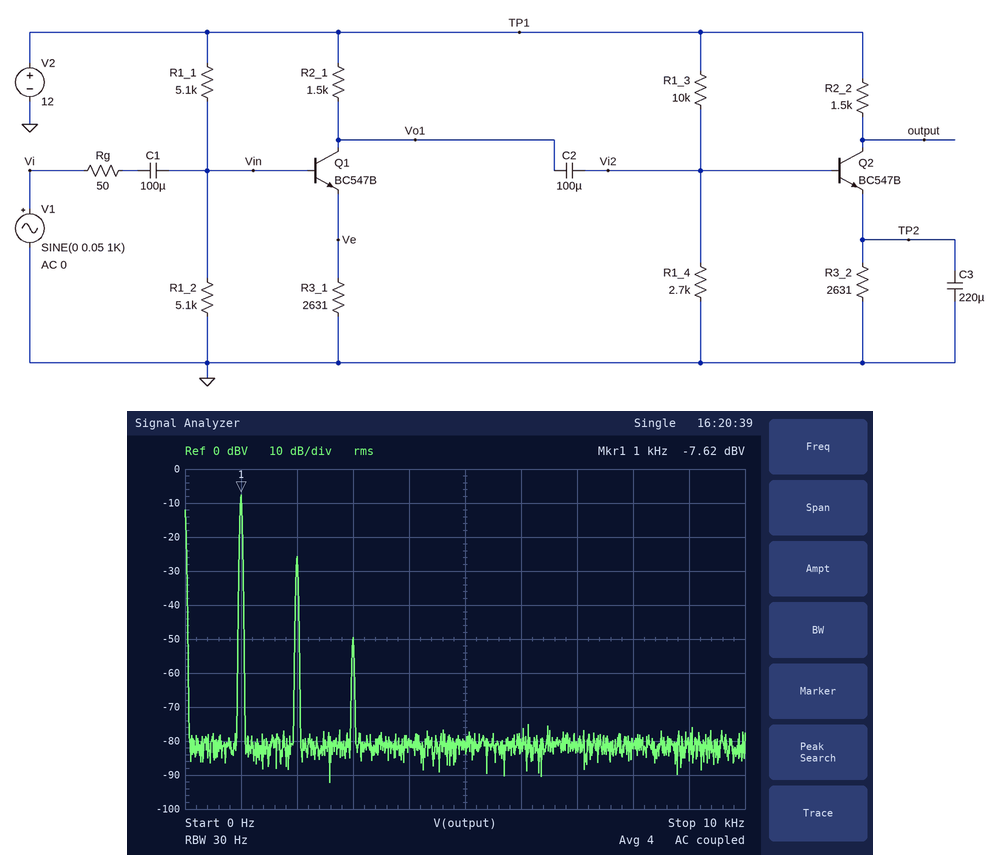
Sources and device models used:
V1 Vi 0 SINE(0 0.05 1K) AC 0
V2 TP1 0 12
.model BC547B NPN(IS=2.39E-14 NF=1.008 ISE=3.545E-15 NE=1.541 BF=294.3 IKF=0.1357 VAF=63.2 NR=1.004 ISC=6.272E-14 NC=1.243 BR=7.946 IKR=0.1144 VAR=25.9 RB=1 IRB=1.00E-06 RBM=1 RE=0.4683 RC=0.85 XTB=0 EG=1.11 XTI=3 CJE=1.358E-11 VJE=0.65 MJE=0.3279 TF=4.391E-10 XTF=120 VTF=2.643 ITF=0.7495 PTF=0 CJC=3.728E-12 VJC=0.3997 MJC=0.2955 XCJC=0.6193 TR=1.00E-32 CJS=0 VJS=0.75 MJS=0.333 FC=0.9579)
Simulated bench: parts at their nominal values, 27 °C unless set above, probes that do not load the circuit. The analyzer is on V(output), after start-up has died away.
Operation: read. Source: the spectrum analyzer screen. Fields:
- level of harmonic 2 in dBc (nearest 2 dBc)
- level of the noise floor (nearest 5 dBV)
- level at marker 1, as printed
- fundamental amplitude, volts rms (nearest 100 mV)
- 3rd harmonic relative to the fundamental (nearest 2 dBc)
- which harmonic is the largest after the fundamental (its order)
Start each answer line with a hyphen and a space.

- -18 dBc
- -80 dBV
- -7.62 dBV
- 400 mV
- -42 dBc
- 2
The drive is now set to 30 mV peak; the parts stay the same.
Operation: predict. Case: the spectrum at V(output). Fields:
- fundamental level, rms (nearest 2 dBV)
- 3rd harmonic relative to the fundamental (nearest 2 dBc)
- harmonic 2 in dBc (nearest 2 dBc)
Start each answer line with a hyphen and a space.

- -12 dBV
- -50 dBc
- -22 dBc
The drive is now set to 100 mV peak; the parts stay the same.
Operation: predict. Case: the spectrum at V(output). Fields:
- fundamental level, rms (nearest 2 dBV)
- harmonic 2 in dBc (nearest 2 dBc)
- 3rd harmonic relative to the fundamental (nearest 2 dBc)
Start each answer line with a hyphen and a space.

- -2 dBV
- -12 dBc
- -30 dBc
